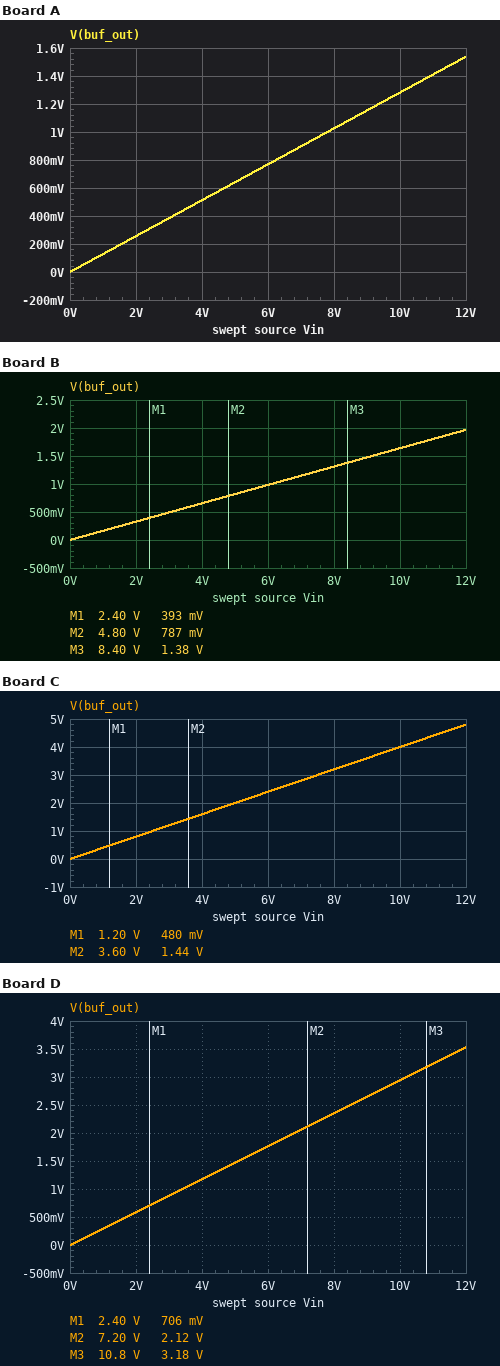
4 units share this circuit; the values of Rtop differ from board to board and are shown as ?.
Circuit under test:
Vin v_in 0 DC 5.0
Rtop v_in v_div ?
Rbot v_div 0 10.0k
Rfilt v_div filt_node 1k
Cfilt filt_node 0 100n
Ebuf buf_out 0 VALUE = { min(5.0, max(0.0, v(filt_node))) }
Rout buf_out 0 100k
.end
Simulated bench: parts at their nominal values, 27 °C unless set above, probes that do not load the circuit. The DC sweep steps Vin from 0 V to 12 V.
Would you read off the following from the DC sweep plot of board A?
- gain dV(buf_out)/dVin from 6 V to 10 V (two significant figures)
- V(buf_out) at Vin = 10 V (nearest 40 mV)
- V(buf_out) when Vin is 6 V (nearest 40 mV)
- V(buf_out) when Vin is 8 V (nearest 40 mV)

0.13 V/V
1.28 V
760 mV
1.04 V
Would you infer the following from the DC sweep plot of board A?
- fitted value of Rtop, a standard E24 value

68 kΩ
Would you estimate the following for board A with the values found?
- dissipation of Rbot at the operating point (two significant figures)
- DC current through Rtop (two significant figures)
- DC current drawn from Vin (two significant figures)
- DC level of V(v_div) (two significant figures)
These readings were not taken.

41 µW
64 µA
64 µA
640 mV
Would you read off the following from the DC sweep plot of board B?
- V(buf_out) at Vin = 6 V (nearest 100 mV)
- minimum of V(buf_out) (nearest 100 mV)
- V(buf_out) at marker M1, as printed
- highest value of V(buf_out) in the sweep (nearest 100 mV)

1.0 V
0 V
393 mV
2.0 V
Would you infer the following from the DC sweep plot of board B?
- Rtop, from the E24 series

51 kΩ
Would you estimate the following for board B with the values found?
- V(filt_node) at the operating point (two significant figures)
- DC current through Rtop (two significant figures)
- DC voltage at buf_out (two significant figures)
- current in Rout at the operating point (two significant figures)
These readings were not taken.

820 mV
82 µA
820 mV
8.2 µA
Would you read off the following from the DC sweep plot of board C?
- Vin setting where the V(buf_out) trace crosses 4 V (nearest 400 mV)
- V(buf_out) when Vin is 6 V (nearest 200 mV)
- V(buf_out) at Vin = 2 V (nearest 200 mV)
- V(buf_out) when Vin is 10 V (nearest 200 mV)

10.0 V
2.4 V
800 mV
4.0 V
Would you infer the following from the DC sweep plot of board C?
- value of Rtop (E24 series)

15 kΩ
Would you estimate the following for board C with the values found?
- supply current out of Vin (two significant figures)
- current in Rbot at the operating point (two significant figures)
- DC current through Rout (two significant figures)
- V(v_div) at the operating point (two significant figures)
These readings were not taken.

200 µA
200 µA
20 µA
2.0 V
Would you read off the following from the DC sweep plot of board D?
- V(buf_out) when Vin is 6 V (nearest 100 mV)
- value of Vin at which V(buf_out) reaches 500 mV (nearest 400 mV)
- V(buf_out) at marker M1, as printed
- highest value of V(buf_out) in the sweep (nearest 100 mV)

1.8 V
1.6 V
706 mV
3.5 V
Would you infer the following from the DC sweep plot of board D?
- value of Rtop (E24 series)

24 kΩ
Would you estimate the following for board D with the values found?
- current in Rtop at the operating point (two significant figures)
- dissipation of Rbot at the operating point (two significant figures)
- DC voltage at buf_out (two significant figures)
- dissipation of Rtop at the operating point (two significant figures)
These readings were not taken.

150 µA
220 µW
1.5 V
520 µW
